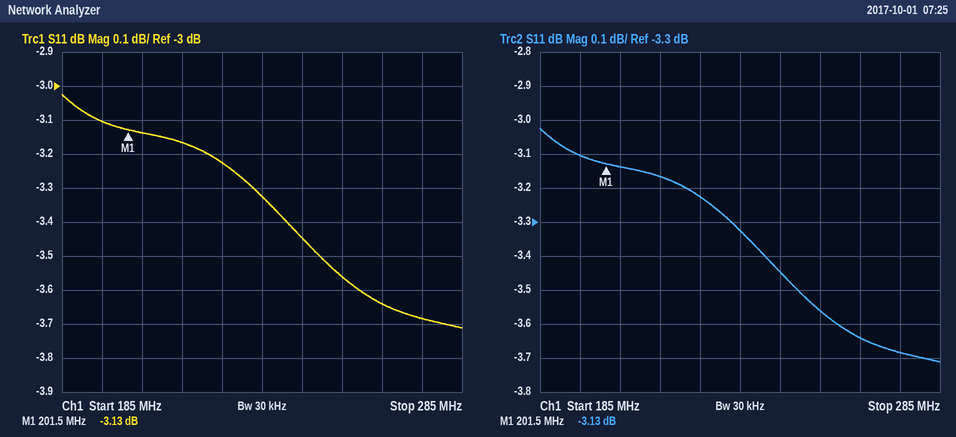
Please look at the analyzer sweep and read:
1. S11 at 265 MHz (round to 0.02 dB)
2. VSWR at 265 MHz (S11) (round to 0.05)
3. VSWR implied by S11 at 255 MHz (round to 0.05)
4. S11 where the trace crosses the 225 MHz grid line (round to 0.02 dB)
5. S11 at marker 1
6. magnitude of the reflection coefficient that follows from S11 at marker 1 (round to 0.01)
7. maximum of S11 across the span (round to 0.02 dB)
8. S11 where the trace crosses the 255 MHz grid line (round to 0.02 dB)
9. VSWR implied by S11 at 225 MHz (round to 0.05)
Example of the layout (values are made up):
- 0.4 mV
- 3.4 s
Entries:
- -3.64 dB
- 4.85
- 4.95
- -3.22 dB
- -3.13 dB
- 0.70
- -3.02 dB
- -3.56 dB
- 5.45
